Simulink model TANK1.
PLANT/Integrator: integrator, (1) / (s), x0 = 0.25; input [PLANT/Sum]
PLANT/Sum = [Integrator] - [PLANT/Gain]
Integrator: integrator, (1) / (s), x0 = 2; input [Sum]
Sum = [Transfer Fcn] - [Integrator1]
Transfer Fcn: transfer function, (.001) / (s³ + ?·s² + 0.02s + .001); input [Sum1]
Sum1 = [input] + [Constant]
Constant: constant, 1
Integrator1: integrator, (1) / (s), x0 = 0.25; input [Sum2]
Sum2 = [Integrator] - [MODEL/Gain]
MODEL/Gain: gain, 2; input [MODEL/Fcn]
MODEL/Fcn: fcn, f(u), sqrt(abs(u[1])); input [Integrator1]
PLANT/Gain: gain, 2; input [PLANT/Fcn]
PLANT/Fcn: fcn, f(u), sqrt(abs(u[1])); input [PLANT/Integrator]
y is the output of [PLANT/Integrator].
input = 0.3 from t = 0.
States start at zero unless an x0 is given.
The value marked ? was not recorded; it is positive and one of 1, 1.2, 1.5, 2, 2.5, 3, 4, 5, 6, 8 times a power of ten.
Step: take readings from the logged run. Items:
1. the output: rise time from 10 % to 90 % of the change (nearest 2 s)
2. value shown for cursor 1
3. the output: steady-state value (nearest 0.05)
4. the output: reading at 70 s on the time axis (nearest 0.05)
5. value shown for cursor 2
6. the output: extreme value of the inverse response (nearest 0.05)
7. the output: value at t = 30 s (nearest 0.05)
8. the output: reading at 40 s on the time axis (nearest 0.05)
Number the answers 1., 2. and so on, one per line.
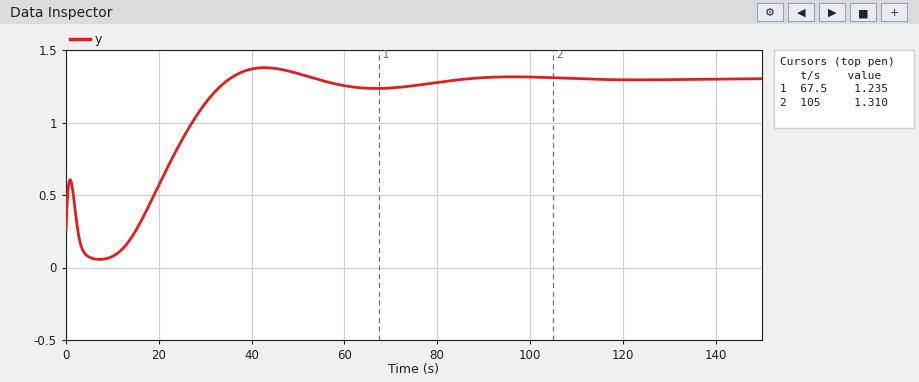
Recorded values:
1. 32 s
2. 1.235
3. 1.30
4. 1.25
5. 1.310
6. 0.05
7. 1.15
8. 1.35
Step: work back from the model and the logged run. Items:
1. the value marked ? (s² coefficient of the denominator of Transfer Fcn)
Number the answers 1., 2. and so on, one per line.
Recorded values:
1. 0.15
